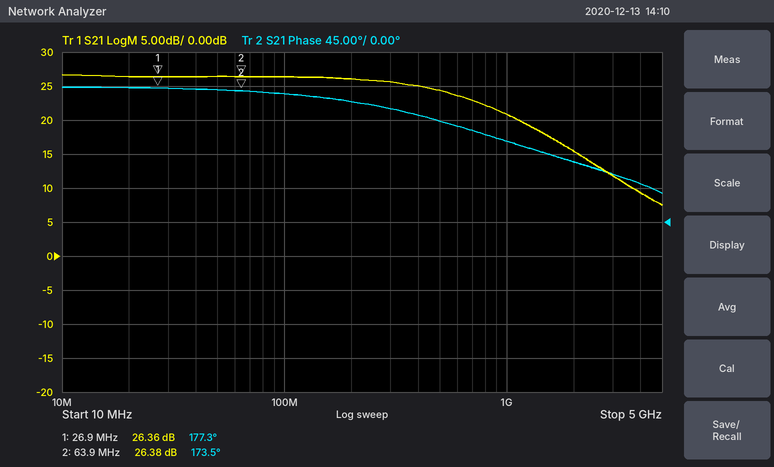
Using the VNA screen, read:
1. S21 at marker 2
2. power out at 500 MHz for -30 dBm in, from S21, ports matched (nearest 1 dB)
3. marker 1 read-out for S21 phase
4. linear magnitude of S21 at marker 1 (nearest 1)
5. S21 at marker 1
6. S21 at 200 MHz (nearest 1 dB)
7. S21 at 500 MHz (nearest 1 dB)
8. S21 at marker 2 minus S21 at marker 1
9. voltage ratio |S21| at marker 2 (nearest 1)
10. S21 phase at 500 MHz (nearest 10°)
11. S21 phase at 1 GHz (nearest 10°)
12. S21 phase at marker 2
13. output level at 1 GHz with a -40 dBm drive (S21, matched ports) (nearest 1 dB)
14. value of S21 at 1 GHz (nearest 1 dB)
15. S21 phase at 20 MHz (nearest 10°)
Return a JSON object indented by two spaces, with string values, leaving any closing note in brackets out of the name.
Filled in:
{
  "S21 at marker 2": "26.38 dB",
  "power out at 500 MHz for -30 dBm in, from S21, ports matched": "-6 dBm",
  "marker 1 read-out for S21 phase": "177.3°",
  "linear magnitude of S21 at marker 1": "21",
  "S21 at marker 1": "26.36 dB",
  "S21 at 200 MHz": "26 dB",
  "S21 at 500 MHz": "24 dB",
  "S21 at marker 2 minus S21 at marker 1": "0.02 dB",
  "voltage ratio |S21| at marker 2": "21",
  "S21 phase at 500 MHz": "130°",
  "S21 phase at 1 GHz": "110°",
  "S21 phase at marker 2": "173.5°",
  "output level at 1 GHz with a -40 dBm drive (S21, matched ports)": "-19 dBm",
  "value of S21 at 1 GHz": "21 dB",
  "S21 phase at 20 MHz": "180°"
}
